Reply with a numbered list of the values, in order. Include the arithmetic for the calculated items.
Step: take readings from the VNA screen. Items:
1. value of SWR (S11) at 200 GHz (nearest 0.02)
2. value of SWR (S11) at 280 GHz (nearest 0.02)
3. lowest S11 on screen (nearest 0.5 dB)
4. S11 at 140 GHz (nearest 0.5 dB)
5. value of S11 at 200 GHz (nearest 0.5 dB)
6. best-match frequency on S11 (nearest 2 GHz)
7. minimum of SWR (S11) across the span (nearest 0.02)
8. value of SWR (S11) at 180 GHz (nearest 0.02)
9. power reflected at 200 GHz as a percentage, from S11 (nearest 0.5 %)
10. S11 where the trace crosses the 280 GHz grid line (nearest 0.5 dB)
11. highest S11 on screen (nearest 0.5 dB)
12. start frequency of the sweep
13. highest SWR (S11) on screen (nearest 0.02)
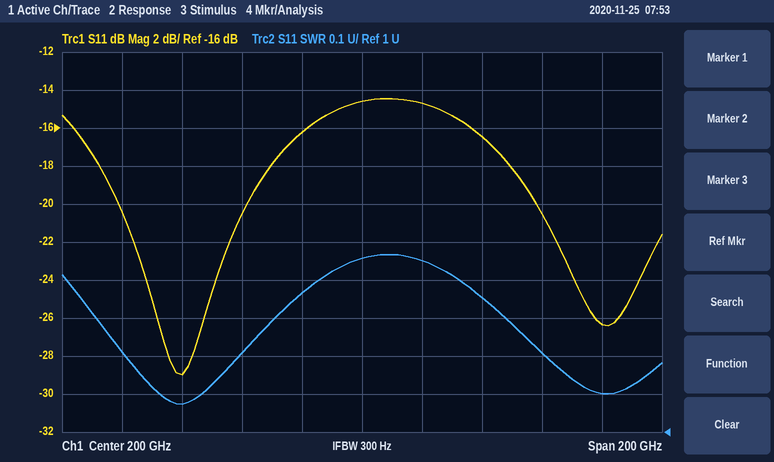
1. 1.46
2. 1.10
3. -29.0 dB
4. -29.0 dB
5. -14.5 dB
6. 140 GHz
7. 1.08
8. 1.36
9. 10^(-14.5/10) ≈ 3.5 %
10. -26.5 dB
11. -14.5 dB
12. 100 GHz
13. 1.46
